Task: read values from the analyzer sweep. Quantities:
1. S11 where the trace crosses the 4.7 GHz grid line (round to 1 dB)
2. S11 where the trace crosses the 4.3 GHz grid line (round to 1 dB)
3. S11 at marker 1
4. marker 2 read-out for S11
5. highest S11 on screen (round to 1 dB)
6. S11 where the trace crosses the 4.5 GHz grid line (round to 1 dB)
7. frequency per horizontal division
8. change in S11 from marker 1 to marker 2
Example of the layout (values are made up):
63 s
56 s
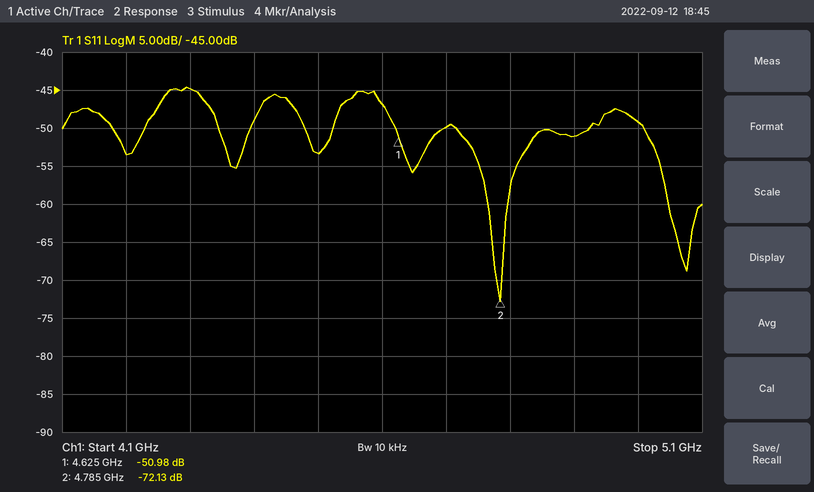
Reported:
-50 dB
-45 dB
-50.98 dB
-72.13 dB
-45 dB
-53 dB
100 MHz
-21.15 dB
